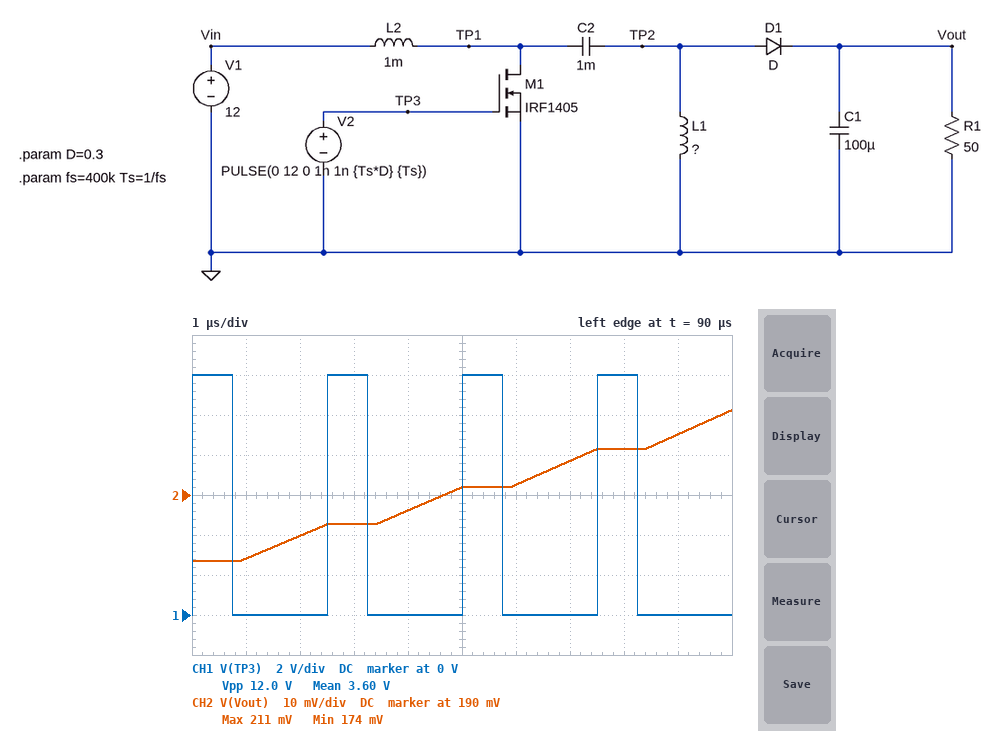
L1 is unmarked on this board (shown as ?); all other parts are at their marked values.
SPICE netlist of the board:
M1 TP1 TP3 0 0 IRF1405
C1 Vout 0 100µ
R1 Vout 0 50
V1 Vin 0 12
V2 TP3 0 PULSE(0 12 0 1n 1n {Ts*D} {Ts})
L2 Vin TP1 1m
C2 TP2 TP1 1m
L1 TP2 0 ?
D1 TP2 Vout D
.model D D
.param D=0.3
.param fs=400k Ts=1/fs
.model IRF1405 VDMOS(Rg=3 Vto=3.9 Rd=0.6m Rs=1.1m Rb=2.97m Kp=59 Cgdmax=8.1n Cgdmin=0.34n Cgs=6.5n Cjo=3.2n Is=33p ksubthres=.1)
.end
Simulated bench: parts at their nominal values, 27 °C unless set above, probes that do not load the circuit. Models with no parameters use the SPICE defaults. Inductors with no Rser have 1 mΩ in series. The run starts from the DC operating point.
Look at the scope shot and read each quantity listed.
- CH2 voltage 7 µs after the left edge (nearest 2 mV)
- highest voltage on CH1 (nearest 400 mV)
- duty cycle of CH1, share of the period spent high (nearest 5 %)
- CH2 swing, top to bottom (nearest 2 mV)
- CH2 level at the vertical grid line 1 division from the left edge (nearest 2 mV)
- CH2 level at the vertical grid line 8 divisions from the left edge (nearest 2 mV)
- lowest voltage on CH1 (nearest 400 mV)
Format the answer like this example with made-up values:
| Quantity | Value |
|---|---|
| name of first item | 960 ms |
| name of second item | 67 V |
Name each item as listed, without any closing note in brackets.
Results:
| Quantity | Value |
|---|---|
| CH2 voltage 7 µs after the left edge | 198 mV |
| highest voltage on CH1 | 12.0 V |
| duty cycle of CH1, share of the period spent high | 30 % |
| CH2 swing, top to bottom | 38 mV |
| CH2 level at the vertical grid line 1 division from the left edge | 174 mV |
| CH2 level at the vertical grid line 8 divisions from the left edge | 202 mV |
| lowest voltage on CH1 | 0 V |
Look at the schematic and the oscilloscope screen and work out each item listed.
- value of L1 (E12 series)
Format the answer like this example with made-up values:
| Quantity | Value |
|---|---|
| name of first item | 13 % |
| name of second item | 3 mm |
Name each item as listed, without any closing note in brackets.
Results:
| Quantity | Value |
|---|---|
| value of L1 | 2.2 mH |
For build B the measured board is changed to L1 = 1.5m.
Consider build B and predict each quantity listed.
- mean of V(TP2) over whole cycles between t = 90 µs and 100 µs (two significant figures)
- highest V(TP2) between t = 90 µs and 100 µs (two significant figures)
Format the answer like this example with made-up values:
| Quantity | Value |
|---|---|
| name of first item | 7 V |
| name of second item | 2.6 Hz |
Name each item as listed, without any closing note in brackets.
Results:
| Quantity | Value |
|---|---|
| mean of V(TP2) over whole cycles between t = 90 µs and 100 µs | -3.4 V |
| highest V(TP2) between t = 90 µs and 100 µs | 1.1 V |
